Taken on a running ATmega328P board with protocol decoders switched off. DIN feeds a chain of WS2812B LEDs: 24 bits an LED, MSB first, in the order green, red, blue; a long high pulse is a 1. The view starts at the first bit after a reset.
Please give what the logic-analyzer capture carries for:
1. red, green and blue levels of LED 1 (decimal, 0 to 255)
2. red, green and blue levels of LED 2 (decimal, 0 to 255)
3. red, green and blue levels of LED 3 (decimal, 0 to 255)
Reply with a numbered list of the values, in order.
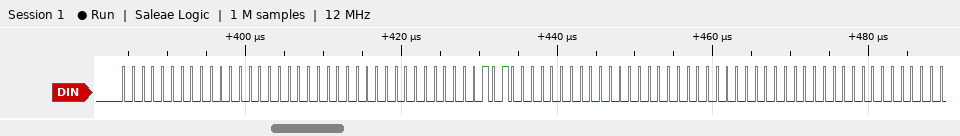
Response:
1. 0, 0, 0
2. 5, 0, 0
3. 0, 0, 0
